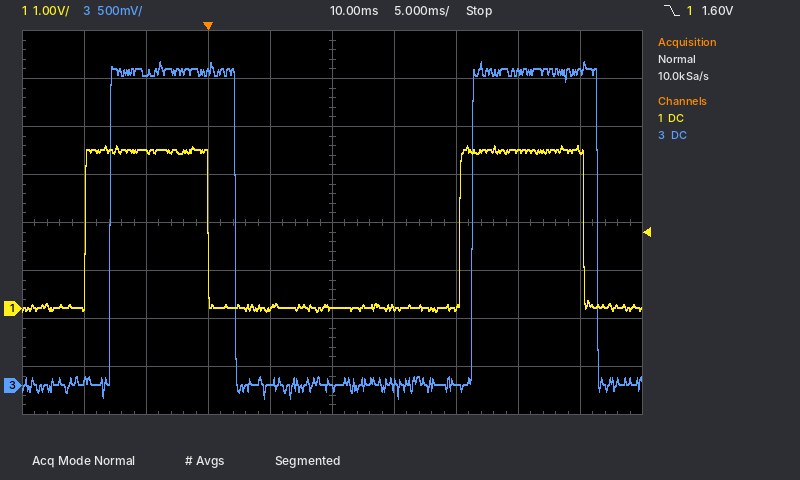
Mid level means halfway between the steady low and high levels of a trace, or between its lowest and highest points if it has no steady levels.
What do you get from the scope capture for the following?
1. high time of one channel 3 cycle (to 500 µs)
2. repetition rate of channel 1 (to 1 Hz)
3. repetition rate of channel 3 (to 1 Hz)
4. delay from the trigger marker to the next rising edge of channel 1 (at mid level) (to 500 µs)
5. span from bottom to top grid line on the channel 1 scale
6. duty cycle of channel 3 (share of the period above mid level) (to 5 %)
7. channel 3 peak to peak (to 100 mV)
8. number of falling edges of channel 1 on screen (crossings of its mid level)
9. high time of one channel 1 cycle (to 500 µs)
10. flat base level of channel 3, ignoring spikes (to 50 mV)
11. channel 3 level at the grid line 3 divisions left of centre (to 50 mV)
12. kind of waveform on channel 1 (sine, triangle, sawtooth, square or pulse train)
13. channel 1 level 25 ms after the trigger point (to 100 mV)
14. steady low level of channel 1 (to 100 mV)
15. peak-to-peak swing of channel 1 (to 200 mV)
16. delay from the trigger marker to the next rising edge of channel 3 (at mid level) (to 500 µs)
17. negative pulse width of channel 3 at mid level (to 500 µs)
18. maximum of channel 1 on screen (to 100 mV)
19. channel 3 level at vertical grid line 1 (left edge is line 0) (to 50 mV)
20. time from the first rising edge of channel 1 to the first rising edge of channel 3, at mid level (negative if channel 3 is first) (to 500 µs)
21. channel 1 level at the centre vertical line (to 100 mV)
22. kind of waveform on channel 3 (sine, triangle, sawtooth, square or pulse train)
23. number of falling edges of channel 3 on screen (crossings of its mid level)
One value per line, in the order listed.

10.0 ms
33 Hz
34 Hz
20.5 ms
8 V
35 %
3.50 V
2
10.0 ms
0 mV
3.25 V
pulse train
3.3 V
0.0 V
3.4 V
21.5 ms
19.0 ms
3.4 V
50 mV
+2.0 ms
0.0 V
pulse train
2
